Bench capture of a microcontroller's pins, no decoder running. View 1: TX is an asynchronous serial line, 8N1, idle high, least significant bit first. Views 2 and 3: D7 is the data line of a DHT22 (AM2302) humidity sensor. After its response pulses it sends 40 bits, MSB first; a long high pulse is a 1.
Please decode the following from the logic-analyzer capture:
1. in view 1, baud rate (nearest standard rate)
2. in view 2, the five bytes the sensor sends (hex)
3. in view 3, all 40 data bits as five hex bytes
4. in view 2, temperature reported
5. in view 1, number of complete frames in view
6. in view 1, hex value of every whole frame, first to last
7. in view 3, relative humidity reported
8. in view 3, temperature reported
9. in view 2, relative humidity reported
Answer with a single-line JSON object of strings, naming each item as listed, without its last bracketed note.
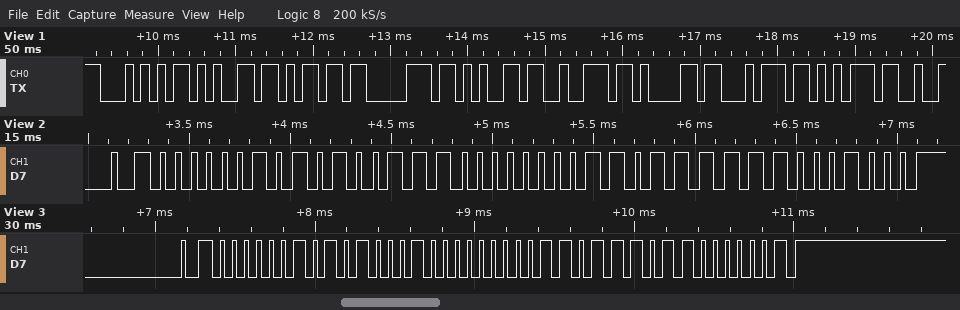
{"in view 1, baud rate": "9600 baud", "in view 2, the five bytes the sensor sends": "02 A7 00 DF 88", "in view 3, all 40 data bits as five hex bytes": "02 A2 00 DD 81", "in view 2, temperature reported": "22.3 °C", "in view 1, number of complete frames in view": "9", "in view 1, hex value of every whole frame, first to last": "0x54 0x65 0x6D 0x70 0x65 0x72 0x61 0x74 0x75", "in view 3, relative humidity reported": "67.4 %", "in view 3, temperature reported": "22.1 °C", "in view 2, relative humidity reported": "67.9 %"}
